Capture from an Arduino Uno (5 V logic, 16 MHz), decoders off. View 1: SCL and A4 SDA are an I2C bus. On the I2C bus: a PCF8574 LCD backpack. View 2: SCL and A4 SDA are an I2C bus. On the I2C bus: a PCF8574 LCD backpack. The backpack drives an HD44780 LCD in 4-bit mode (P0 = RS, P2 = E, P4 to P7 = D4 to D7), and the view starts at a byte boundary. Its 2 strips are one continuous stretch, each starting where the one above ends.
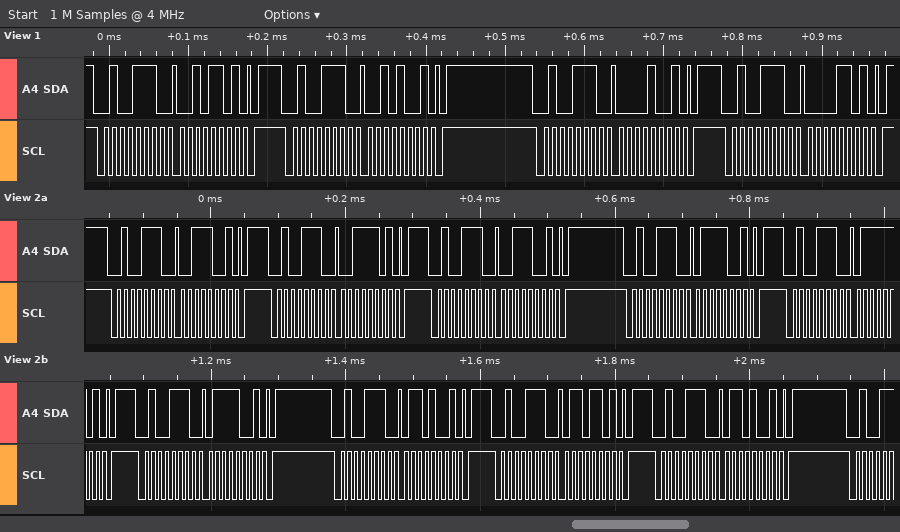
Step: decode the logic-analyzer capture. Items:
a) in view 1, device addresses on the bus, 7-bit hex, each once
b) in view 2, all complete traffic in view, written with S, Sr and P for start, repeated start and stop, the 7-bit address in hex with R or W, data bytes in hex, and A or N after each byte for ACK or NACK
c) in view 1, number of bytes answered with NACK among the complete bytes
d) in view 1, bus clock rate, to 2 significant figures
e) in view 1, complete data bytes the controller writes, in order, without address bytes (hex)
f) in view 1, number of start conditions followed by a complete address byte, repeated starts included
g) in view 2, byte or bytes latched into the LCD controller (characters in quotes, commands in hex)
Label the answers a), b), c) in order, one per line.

a) 0x27
b) S 27W A 39 A P S 27W A 3D A P S 27W A 39 A P S 27W A 79 A P S 27W A 7D A P S 27W A 79 A P S 27W A 69 A P S 27W A 6D A P S 27W A 69 A P
c) 0
d) 100 kHz
e) 2D 29 09 0D
f) 4
g) '7'
